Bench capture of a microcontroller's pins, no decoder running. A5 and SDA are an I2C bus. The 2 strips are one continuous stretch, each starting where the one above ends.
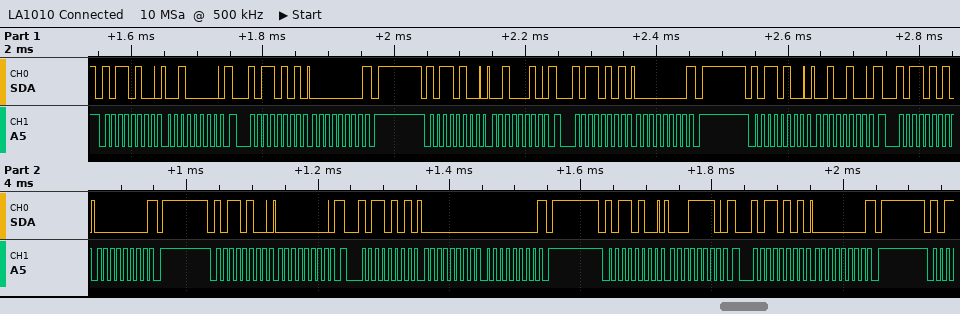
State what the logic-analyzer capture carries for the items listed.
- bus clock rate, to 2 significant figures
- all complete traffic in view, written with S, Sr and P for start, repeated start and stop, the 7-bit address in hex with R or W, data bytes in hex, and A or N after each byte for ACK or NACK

100 kHz
S 5AW A 20 A Sr 5AR A 00 N P S 5AW A 22 A Sr 5AR A 00 N P S 5AW A 24 A Sr 5AR A 00 N P S 5AW A 00 A Sr 5AR A 00 A 00 N P S 5AW A 1E A Sr 5AR A 00 N P
